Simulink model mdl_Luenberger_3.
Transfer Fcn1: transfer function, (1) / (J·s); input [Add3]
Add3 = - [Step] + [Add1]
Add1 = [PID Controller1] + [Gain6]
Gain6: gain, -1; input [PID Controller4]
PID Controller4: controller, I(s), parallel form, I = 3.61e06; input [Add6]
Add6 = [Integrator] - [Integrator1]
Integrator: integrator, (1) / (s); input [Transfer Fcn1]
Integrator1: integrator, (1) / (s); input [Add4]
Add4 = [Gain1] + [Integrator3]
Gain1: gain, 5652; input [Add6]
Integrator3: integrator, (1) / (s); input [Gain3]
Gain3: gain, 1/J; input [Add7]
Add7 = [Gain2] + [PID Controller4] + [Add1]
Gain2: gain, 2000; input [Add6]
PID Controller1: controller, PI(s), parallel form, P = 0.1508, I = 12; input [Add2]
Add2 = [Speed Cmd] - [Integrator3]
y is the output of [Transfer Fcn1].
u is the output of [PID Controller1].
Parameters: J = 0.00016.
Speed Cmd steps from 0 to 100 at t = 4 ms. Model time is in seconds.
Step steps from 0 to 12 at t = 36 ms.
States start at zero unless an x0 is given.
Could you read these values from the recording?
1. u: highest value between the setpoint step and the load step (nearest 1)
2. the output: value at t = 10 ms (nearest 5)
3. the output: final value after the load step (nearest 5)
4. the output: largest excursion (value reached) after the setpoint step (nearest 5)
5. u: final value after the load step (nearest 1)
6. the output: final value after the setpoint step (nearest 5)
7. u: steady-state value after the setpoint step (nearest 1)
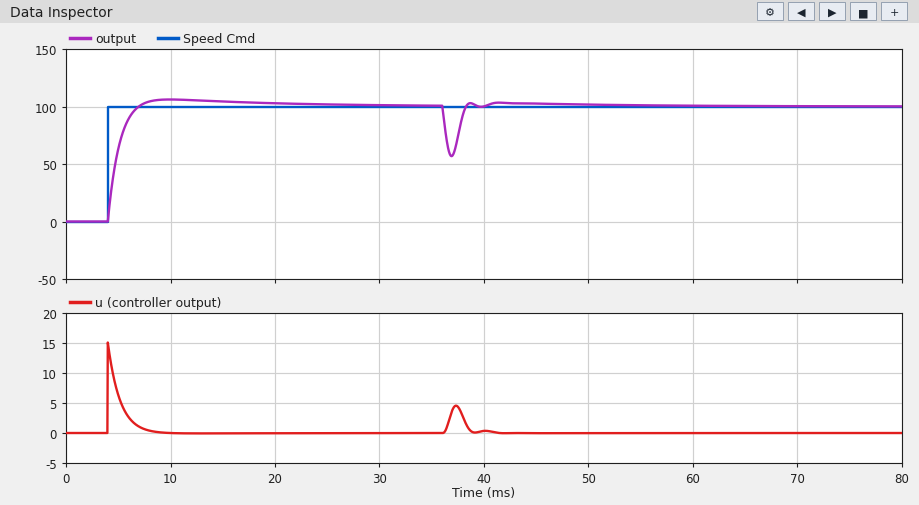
15
105
100
105
0
100
0
